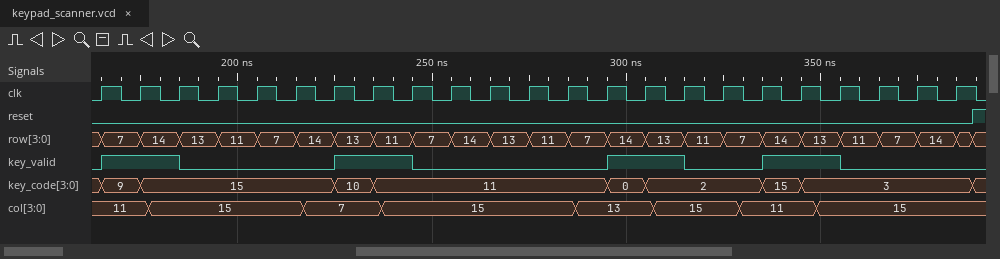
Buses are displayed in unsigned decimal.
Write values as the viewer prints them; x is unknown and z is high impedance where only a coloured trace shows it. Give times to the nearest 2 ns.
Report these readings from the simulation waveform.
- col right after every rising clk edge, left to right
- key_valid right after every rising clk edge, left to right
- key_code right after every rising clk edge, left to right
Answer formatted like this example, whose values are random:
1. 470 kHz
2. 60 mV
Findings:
1. 11, 11, 15, 15, 15, 15, 7, 7, 15, 15, 15, 15, 15, 13, 13, 15, 15, 11, 11, 15, 15, 15, 15
2. 1 1 0 0 0 0 1 1 0 0 0 0 0 1 1 0 0 1 1 0 0 0 0
3. 9, 15, 15, 15, 15, 15, 10, 11, 11, 11, 11, 11, 11, 0, 2, 2, 2, 15, 3, 3, 3, 3, 3
